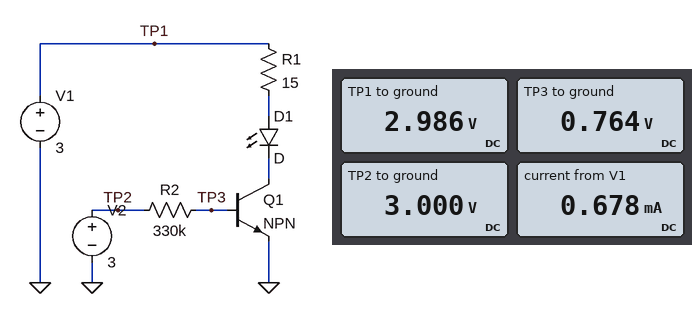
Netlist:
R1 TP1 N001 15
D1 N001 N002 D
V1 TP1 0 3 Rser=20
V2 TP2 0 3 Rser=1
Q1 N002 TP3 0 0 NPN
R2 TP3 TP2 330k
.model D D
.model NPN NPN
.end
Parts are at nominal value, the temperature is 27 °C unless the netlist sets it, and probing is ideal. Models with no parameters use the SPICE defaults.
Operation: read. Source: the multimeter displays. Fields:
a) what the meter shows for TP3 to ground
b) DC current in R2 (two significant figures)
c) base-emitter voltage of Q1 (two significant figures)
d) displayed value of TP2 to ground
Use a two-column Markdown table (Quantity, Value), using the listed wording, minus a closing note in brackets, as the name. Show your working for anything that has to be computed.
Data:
| Quantity | Value |
|---|---|
| what the meter shows for TP3 to ground | 0.764 V |
| DC current in R2 | (3 V - 764 mV) / 330 kΩ = 6.8 µA |
| base-emitter voltage of Q1 | 764 mV = 760 mV |
| displayed value of TP2 to ground | 3.000 V |
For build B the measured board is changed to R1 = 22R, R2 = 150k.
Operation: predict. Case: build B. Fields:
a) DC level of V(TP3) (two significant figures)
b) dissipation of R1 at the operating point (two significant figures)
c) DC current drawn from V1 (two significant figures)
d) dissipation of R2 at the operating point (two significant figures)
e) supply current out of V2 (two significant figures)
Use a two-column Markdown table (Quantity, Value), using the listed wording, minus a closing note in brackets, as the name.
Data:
| Quantity | Value |
|---|---|
| DC level of V(TP3) | 780 mV |
| dissipation of R1 at the operating point | 48 µW |
| DC current drawn from V1 | 1.5 mA |
| dissipation of R2 at the operating point | 33 µW |
| supply current out of V2 | 15 µA |
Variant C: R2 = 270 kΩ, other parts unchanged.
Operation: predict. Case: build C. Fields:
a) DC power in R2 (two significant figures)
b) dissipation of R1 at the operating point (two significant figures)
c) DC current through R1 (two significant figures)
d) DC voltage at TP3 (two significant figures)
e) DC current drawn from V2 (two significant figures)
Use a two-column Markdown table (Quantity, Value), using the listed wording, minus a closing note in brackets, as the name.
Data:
| Quantity | Value |
|---|---|
| DC power in R2 | 18 µW |
| dissipation of R1 at the operating point | 10 µW |
| DC current through R1 | 830 µA |
| DC voltage at TP3 | 770 mV |
| DC current drawn from V2 | 8.3 µA |
